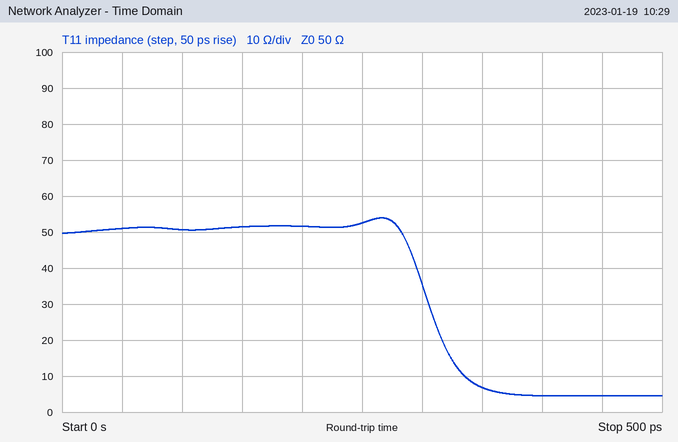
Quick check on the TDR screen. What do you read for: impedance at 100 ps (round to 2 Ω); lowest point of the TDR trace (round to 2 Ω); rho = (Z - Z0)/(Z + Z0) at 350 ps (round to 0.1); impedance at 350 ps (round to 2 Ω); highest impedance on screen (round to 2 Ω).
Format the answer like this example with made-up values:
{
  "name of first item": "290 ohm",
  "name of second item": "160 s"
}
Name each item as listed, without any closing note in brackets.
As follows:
{
  "impedance at 100 ps": "50 Ω",
  "lowest point of the TDR trace": "4 Ω",
  "rho = (Z - Z0)/(Z + Z0) at 350 ps": "-0.8",
  "impedance at 350 ps": "6 Ω",
  "highest impedance on screen": "54 Ω"
}
